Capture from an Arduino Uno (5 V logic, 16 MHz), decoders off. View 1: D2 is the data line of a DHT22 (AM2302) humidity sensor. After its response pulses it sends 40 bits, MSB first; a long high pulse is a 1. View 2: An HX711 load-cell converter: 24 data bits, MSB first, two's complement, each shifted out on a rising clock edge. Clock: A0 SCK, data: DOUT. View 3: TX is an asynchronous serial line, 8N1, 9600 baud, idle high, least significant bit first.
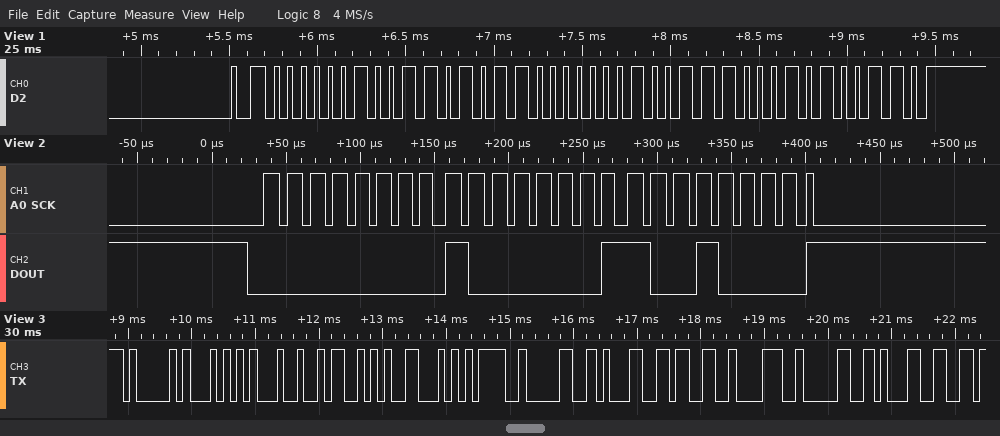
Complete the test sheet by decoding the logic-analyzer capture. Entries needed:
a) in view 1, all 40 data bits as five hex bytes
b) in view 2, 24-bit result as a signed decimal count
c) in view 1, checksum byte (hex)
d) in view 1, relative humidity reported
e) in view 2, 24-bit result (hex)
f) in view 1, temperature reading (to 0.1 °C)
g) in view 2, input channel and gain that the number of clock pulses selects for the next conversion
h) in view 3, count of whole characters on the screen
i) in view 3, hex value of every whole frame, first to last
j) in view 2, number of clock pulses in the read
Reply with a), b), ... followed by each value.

a) 02 6B 01 38 A6
b) 33168
c) 0xA6
d) 61.9 %
e) 0x008190
f) 31.2 °C
g) channel A, gain 128
h) 12
i) 41 54 24 53 46 3D 30 31 33 38 30 31
j) 25
